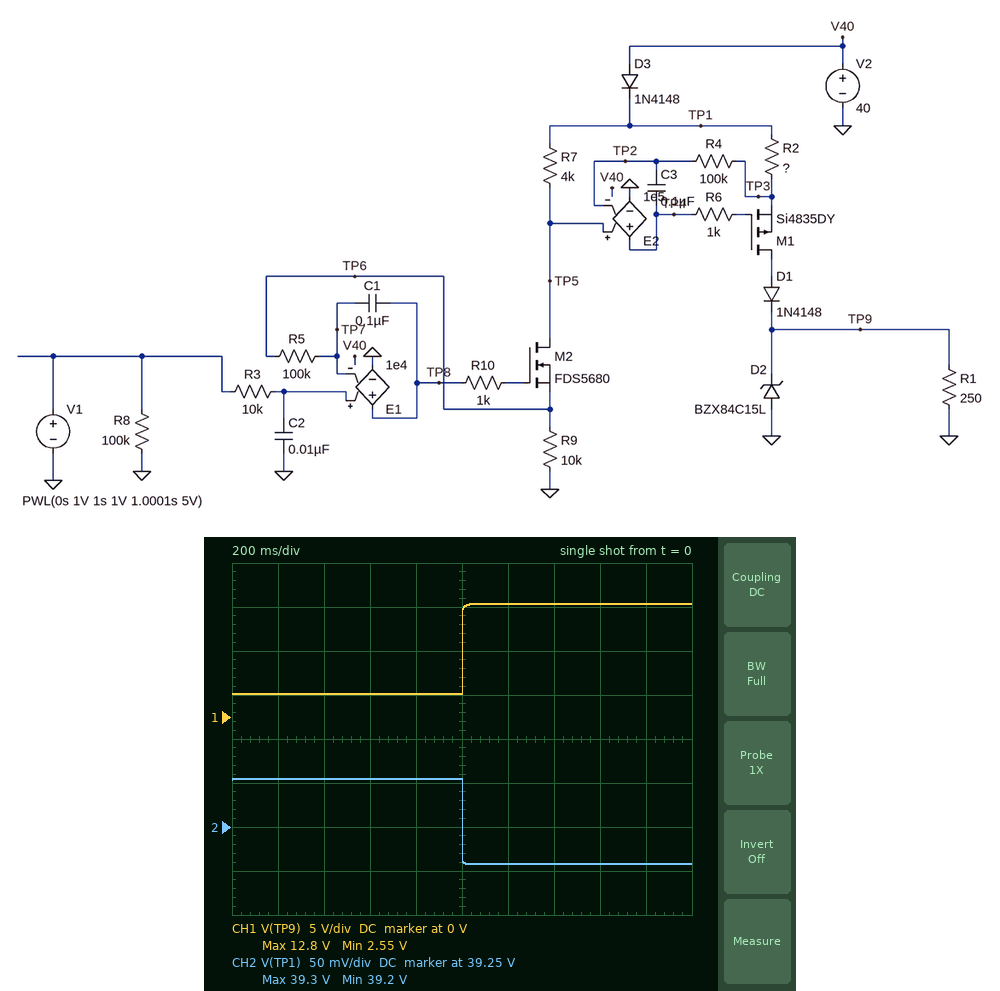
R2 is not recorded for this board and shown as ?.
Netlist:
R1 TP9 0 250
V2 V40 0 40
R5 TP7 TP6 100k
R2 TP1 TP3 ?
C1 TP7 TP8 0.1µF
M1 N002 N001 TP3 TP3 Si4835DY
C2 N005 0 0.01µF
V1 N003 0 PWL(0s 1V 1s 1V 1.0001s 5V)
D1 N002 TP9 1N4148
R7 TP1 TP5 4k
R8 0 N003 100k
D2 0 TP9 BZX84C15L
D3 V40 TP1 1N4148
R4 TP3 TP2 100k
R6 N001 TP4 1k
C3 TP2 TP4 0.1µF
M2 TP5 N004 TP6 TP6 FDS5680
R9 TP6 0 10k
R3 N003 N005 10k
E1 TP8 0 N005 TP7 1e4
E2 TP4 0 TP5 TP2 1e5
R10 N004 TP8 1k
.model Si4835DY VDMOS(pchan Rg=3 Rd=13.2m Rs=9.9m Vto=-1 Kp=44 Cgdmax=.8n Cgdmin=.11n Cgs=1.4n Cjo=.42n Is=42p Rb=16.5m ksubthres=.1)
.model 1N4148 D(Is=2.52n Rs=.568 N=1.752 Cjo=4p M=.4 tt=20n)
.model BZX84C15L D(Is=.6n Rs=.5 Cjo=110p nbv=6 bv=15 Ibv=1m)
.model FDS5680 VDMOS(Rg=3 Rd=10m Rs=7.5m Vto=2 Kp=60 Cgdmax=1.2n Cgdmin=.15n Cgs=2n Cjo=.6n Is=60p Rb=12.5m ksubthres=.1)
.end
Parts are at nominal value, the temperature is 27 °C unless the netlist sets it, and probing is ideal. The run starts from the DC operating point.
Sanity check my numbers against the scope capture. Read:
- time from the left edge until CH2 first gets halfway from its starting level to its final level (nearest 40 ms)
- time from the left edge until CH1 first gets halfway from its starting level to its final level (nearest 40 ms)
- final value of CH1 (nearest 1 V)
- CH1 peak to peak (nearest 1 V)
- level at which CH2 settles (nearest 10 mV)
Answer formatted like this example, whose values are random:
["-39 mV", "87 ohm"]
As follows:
["1.00 s", "1.00 s", "13 V", "10 V", "39.21 V"]
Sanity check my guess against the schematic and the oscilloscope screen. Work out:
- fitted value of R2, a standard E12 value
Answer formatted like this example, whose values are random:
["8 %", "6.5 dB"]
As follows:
["39 Ω"]
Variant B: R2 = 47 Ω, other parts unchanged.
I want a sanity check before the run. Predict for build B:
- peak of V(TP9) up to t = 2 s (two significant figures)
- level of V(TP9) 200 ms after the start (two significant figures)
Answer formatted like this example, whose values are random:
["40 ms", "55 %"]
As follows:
["11 V", "2.1 V"]
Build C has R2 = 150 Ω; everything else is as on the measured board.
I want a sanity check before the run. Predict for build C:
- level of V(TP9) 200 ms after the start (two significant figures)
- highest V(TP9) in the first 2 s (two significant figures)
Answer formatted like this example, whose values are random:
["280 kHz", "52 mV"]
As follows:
["670 mV", "3.3 V"]
